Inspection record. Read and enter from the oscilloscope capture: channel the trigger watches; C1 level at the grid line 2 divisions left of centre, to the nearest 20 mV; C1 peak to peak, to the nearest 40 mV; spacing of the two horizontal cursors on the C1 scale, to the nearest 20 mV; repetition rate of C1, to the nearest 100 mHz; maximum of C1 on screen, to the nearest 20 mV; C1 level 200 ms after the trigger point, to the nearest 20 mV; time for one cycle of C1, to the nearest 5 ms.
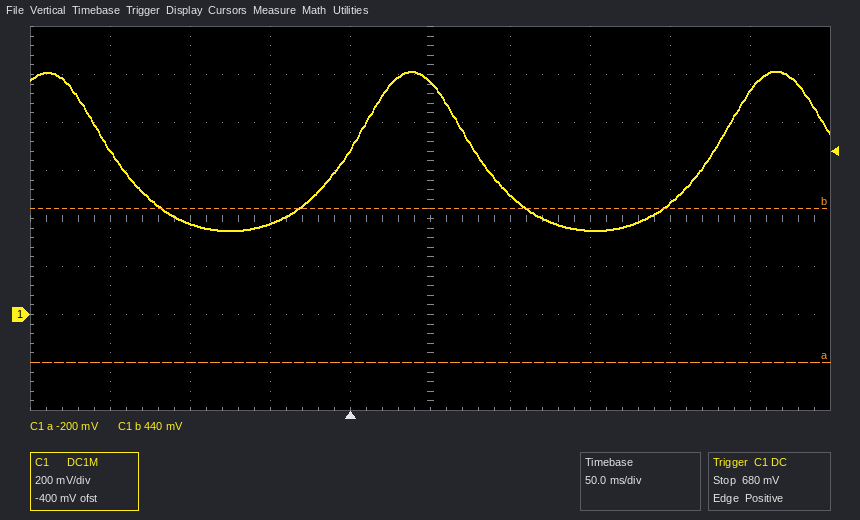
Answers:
C1
380 mV
680 mV
640 mV
4.4 Hz
1.02 V
460 mV
225 ms
